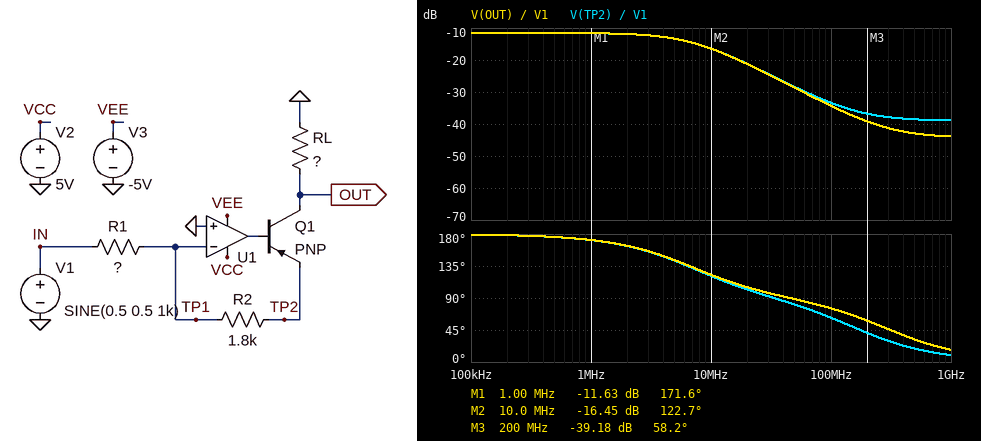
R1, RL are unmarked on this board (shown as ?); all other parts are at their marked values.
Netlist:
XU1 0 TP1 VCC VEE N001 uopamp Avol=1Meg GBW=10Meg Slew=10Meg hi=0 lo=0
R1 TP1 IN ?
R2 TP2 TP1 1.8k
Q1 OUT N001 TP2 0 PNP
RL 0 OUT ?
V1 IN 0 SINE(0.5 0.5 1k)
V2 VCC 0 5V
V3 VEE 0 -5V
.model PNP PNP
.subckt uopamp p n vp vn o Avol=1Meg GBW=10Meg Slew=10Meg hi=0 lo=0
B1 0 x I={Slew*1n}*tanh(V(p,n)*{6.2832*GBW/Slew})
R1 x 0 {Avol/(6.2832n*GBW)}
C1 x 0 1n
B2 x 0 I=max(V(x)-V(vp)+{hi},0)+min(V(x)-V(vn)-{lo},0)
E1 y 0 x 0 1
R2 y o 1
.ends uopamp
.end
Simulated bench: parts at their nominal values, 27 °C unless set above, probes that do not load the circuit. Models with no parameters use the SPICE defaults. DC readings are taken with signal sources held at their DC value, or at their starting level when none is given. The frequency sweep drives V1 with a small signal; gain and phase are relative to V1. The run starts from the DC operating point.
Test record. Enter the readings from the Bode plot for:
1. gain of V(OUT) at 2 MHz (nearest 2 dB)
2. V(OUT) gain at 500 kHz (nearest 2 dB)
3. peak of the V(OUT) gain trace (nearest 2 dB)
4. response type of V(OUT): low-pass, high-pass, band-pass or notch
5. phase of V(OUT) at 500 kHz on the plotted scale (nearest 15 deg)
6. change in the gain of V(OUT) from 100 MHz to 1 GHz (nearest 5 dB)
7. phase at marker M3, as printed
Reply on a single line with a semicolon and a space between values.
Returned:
-12 dB; -12 dB; -12 dB; low-pass; 180 deg; -10 dB; 58.2 deg
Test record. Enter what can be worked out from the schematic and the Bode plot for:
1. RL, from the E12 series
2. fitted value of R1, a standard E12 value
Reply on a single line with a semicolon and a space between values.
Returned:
390 Ω; 6.8 kΩ
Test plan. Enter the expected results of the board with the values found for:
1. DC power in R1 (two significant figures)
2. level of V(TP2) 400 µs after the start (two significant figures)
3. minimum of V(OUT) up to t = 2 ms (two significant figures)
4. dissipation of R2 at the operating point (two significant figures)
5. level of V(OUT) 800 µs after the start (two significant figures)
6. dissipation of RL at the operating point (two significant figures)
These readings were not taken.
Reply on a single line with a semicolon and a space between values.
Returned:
37 µW; -210 mV; -270 mV; 9.7 µW; -9.4 mV; 48 µW
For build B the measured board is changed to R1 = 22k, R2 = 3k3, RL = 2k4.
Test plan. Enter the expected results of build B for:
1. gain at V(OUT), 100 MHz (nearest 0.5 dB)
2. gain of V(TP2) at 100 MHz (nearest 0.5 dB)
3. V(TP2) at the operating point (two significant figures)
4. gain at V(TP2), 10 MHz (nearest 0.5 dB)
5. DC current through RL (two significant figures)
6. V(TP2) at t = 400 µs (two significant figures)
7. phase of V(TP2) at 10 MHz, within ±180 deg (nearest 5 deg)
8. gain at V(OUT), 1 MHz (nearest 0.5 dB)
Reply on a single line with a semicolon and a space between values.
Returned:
-34.5 dB; -32.0 dB; -75 mV; -20.5 dB; 35 µA; -120 mV; 115 deg; -16.5 dB
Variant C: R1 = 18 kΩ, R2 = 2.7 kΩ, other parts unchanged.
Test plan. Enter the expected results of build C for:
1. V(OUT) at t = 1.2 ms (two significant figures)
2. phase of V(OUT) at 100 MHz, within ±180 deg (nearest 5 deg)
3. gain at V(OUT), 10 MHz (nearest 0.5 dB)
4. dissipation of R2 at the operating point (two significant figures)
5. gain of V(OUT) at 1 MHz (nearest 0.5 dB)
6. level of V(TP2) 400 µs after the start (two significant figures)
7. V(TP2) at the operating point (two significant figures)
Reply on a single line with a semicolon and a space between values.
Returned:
-150 mV; 70 deg; -21.5 dB; 2.1 µW; -16.5 dB; -120 mV; -75 mV
